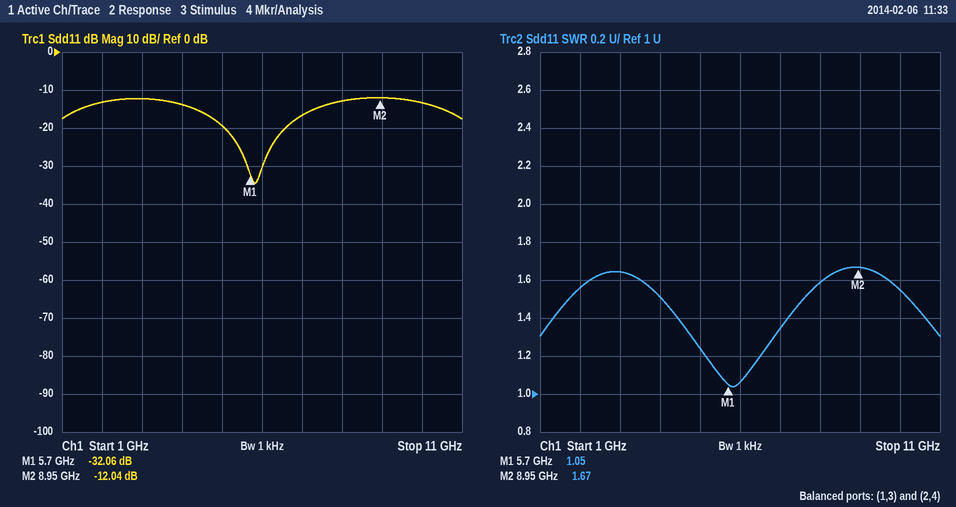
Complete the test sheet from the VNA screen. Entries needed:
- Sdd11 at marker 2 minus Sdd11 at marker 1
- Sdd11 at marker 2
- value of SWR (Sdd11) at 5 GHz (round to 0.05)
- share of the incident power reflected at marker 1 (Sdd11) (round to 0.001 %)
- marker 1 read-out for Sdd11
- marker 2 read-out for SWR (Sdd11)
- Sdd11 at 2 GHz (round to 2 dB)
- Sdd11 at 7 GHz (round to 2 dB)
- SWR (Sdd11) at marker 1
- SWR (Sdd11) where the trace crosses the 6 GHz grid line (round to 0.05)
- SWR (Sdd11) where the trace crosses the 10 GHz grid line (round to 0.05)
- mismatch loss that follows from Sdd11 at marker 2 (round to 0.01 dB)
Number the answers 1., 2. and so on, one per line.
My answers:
1. 20.02 dB
2. -12.04 dB
3. 1.25
4. 0.062 %
5. -32.06 dB
6. 1.67
7. -14 dB
8. -16 dB
9. 1.05
10. 1.05
11. 1.55
12. 0.28 dB
